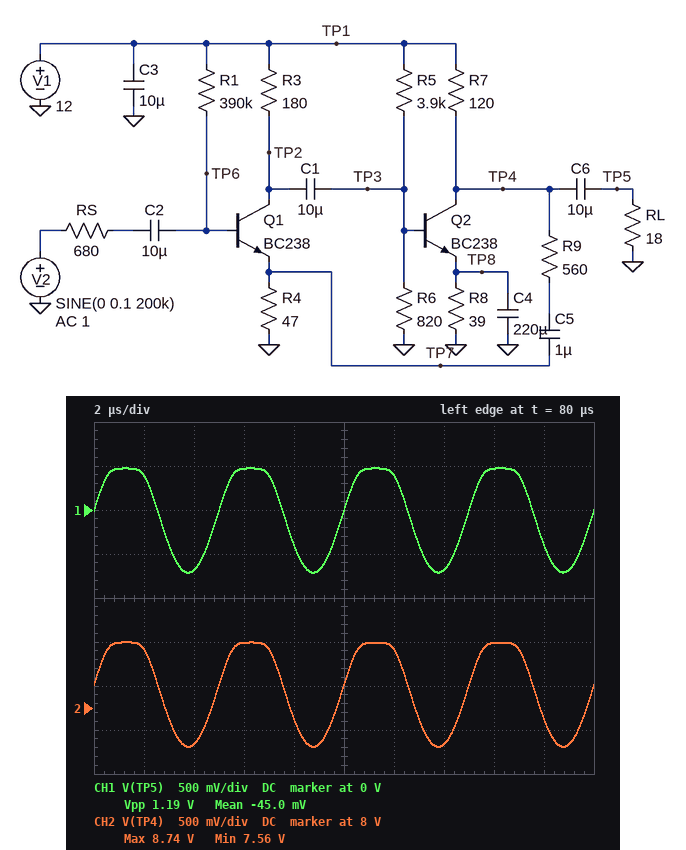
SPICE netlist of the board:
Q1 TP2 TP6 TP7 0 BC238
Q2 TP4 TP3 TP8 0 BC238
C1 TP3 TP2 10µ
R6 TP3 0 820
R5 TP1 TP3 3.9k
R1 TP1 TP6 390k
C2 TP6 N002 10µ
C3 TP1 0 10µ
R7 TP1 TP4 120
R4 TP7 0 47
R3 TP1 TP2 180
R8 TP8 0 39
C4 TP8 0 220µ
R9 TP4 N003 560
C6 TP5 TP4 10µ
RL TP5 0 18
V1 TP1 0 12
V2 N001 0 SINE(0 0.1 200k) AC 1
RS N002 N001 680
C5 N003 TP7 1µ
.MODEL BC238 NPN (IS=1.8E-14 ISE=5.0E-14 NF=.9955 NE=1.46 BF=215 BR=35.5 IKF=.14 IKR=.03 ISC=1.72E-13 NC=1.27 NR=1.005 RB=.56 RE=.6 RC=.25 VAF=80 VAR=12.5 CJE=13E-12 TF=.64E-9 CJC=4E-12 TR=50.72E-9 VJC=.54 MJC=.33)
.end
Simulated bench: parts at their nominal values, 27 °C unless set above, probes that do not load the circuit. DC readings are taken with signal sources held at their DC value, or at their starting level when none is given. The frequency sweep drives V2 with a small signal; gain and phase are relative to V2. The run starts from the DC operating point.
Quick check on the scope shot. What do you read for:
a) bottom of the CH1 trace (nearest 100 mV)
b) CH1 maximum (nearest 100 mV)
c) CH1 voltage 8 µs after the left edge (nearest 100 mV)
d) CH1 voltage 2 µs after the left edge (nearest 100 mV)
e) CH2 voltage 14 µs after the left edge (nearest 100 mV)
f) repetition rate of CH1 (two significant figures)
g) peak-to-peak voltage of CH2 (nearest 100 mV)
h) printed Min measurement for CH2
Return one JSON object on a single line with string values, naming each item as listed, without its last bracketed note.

{"bottom of the CH1 trace": "-700 mV", "CH1 maximum": "500 mV", "CH1 voltage 8 µs after the left edge": "-400 mV", "CH1 voltage 2 µs after the left edge": "400 mV", "CH2 voltage 14 µs after the left edge": "7.6 V", "repetition rate of CH1": "200 kHz", "peak-to-peak voltage of CH2": "1.2 V", "printed Min measurement for CH2": "7.56 V"}
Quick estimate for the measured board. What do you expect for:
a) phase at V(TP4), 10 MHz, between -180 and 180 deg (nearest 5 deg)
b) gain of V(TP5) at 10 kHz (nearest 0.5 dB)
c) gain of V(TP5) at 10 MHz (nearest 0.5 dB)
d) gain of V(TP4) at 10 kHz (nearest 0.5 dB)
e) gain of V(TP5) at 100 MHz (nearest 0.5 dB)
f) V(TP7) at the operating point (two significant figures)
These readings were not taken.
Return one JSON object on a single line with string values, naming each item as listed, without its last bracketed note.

{"phase at V(TP4), 10 MHz, between -180 and 180 deg": "-80 deg", "gain of V(TP5) at 10 kHz": "17.0 dB", "gain of V(TP5) at 10 MHz": "13.5 dB", "gain of V(TP4) at 10 kHz": "17.0 dB", "gain of V(TP5) at 100 MHz": "-20.5 dB", "V(TP7) at the operating point": "260 mV"}
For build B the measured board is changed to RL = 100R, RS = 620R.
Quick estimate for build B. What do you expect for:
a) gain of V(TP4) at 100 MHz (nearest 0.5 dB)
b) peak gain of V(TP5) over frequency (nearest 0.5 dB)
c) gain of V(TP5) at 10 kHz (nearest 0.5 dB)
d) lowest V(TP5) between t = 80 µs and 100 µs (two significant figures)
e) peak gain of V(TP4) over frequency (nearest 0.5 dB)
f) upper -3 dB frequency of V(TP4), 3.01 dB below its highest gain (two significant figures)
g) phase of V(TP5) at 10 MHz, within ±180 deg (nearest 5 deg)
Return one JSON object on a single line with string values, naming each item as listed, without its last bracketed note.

{"gain of V(TP4) at 100 MHz": "-10.0 dB", "peak gain of V(TP5) over frequency": "23.5 dB", "gain of V(TP5) at 10 kHz": "20.5 dB", "lowest V(TP5) between t = 80 µs and 100 µs": "-1.0 V", "peak gain of V(TP4) over frequency": "28.5 dB", "upper -3 dB frequency of V(TP4), 3.01 dB below its highest gain": "190 Hz", "phase of V(TP5) at 10 MHz, within ±180 deg": "-45 deg"}
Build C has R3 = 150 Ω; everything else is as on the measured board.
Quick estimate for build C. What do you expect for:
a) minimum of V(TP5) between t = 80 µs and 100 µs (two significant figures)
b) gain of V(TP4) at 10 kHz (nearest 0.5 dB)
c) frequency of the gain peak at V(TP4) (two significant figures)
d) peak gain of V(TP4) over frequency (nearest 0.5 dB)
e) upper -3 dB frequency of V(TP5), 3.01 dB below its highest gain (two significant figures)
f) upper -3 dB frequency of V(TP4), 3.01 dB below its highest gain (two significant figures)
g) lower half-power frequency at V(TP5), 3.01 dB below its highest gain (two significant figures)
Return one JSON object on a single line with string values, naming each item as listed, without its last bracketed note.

{"minimum of V(TP5) between t = 80 µs and 100 µs": "-690 mV", "gain of V(TP4) at 10 kHz": "16.5 dB", "frequency of the gain peak at V(TP4)": "88 Hz", "peak gain of V(TP4) over frequency": "27.0 dB", "upper -3 dB frequency of V(TP5), 3.01 dB below its highest gain": "9.5 MHz", "upper -3 dB frequency of V(TP4), 3.01 dB below its highest gain": "170 Hz", "lower half-power frequency at V(TP5), 3.01 dB below its highest gain": "610 Hz"}
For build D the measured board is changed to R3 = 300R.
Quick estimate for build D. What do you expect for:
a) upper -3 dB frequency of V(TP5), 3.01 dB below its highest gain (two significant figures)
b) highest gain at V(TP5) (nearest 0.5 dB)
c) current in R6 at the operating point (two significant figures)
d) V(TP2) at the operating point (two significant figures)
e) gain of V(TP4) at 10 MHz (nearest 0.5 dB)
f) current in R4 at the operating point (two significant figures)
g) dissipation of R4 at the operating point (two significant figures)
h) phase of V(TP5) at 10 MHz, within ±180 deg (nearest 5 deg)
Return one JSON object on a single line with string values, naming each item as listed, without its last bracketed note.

{"upper -3 dB frequency of V(TP5), 3.01 dB below its highest gain": "8.9 MHz", "highest gain at V(TP5)": "18.0 dB", "current in R6 at the operating point": "2.4 mA", "V(TP2) at the operating point": "10 V", "gain of V(TP4) at 10 MHz": "14.0 dB", "current in R4 at the operating point": "5.5 mA", "dissipation of R4 at the operating point": "1.4 mW", "phase of V(TP5) at 10 MHz, within ±180 deg": "-85 deg"}
